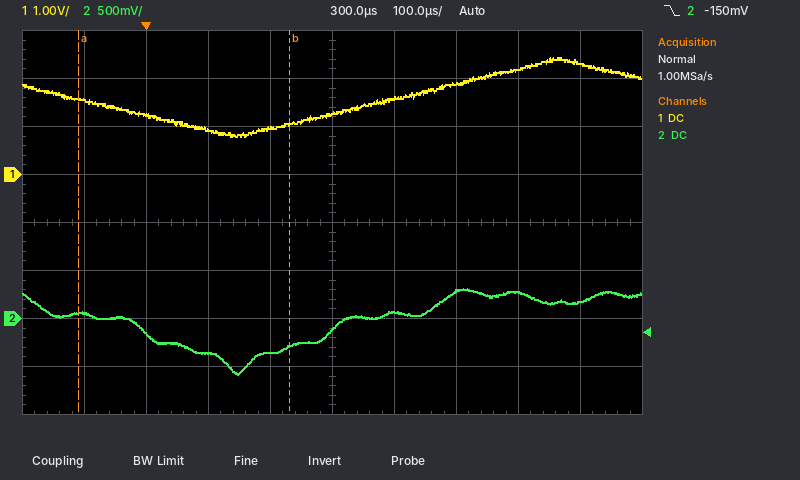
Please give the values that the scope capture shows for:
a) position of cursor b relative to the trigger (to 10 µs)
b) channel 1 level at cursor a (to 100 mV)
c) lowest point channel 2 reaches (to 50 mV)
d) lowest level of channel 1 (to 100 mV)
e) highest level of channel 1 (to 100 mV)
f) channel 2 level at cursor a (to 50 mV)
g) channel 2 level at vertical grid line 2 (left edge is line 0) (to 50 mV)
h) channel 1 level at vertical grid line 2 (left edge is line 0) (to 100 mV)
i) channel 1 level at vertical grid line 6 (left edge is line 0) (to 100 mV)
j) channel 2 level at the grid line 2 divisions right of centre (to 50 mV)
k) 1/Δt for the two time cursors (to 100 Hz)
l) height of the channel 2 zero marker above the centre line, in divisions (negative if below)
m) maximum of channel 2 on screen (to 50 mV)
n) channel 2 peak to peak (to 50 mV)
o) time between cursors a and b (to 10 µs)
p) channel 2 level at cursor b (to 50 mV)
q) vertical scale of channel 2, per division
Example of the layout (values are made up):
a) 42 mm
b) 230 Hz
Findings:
a) +230 µs
b) 1.6 V
c) -600 mV
d) 800 mV
e) 2.4 V
f) 50 mV
g) -150 mV
h) 1.2 V
i) 1.6 V
j) 300 mV
k) 2.9 kHz
l) -2.0 div
m) 300 mV
n) 900 mV
o) 340 µs
p) -300 mV
q) 500 mV
